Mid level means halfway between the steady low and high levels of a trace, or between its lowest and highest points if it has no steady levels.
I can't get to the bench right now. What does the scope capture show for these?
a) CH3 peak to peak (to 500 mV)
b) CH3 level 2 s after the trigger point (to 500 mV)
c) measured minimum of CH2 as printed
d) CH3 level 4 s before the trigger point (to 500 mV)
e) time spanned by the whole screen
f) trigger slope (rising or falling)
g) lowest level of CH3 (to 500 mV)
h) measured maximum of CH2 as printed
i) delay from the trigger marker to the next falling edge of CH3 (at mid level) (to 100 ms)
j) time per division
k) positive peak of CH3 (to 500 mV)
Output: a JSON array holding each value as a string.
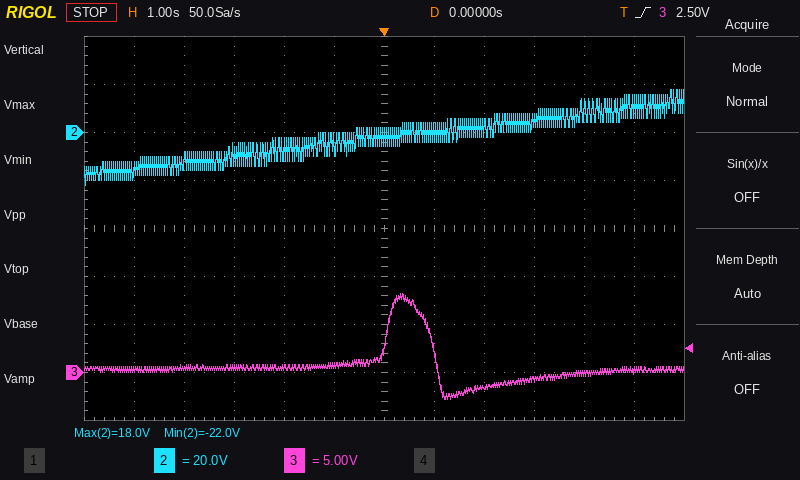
["11.0 V", "-1.5 V", "-22.0 V", "500 mV", "12 s", "rising", "-3.0 V", "18.0 V", "1.0 s", "1 s", "8.0 V"]
